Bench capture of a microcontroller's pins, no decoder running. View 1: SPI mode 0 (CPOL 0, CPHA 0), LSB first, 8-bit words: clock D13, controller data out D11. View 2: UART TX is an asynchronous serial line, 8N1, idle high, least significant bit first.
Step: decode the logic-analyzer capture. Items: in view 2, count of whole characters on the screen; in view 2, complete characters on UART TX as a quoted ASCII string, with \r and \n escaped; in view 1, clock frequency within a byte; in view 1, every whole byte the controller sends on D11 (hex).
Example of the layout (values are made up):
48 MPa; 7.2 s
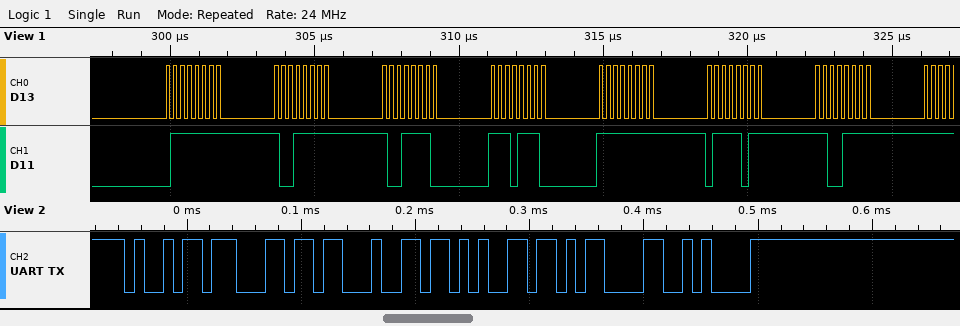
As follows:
6; "ilde\r\n"; 4 MHz; FE F9 79 77 FF DE F3
